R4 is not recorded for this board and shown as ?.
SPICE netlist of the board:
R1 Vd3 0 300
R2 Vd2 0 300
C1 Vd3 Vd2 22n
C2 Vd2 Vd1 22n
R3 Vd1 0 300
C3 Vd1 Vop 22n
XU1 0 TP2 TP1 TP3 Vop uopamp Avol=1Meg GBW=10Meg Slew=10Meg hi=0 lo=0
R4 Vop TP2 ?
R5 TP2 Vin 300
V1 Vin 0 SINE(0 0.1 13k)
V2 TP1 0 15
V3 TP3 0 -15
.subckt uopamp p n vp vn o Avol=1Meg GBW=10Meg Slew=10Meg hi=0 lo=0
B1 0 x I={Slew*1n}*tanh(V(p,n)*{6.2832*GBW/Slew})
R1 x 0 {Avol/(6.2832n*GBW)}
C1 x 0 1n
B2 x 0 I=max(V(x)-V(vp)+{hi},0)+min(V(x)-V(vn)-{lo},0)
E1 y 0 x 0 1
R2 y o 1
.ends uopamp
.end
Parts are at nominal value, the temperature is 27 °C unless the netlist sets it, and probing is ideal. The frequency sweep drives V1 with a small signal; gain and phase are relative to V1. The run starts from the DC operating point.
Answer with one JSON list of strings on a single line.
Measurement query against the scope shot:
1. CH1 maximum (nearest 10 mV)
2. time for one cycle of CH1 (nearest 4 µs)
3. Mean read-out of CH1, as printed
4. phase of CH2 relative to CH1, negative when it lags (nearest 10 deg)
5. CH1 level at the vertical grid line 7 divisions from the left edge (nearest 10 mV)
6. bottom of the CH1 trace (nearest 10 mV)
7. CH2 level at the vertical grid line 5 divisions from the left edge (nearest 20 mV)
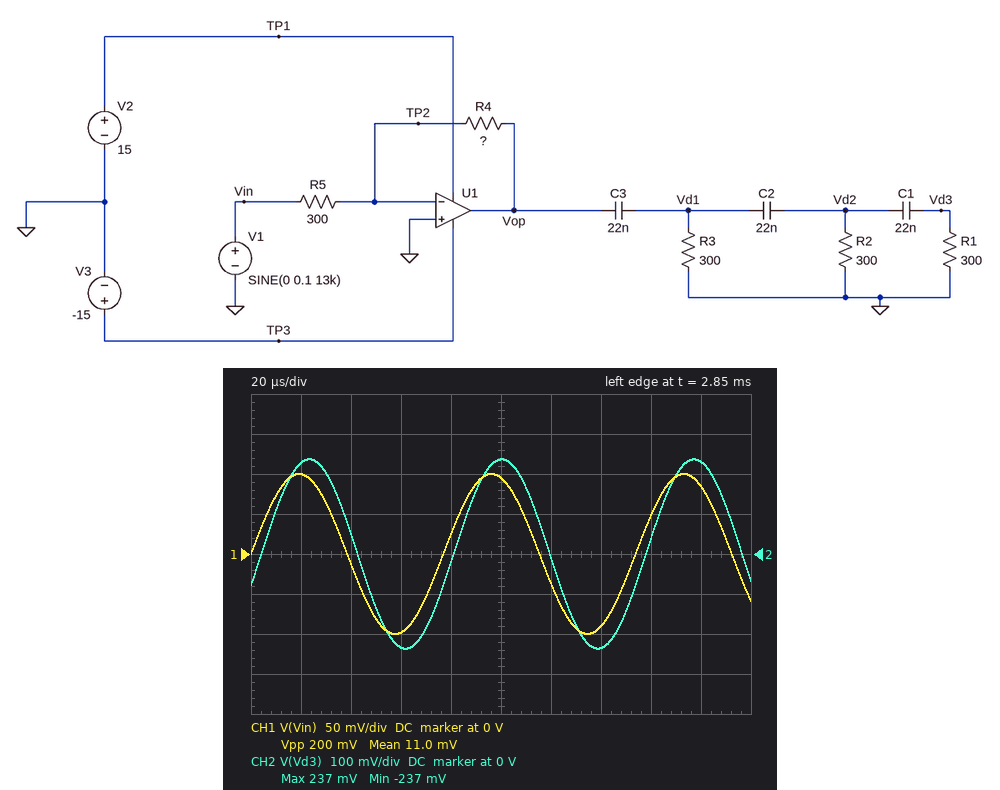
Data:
["100 mV", "76 µs", "11.0 mV", "-20 deg", "-90 mV", "-100 mV", "240 mV"]
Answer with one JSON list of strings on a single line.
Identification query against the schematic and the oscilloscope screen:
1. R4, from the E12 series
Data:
["12 kΩ"]
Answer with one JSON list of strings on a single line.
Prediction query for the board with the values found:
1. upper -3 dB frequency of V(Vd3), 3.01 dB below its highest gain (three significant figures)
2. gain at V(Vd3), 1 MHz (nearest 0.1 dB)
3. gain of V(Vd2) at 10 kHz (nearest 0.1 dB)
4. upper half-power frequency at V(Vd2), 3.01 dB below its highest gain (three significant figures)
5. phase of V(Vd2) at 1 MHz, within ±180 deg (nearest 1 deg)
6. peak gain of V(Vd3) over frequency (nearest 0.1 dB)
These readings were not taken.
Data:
["433 kHz", "19.4 dB", "11.4 dB", "428 kHz", "110 deg", "28.5 dB"]
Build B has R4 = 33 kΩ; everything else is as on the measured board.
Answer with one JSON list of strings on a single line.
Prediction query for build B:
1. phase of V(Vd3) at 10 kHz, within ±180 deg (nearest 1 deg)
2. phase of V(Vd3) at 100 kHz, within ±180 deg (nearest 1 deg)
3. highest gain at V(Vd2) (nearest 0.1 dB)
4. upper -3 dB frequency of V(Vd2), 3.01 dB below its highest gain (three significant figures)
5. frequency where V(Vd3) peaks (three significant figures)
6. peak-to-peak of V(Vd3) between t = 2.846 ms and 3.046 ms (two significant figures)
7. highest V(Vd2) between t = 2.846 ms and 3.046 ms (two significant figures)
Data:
["-7 deg", "-165 deg", "33.5 dB", "249 kHz", "107 kHz", "1.3 V", "1.4 V"]
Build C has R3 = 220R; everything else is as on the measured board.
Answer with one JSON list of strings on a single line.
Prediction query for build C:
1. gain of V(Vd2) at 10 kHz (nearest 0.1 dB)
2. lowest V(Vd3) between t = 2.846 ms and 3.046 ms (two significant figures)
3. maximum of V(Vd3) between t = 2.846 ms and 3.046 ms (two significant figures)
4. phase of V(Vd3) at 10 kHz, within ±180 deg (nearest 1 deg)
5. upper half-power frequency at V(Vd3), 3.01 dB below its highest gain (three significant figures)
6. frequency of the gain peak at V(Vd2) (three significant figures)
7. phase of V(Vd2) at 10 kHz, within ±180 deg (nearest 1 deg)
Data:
["9.6 dB", "-200 mV", "200 mV", "4 deg", "440 kHz", "174 kHz", "-64 deg"]
